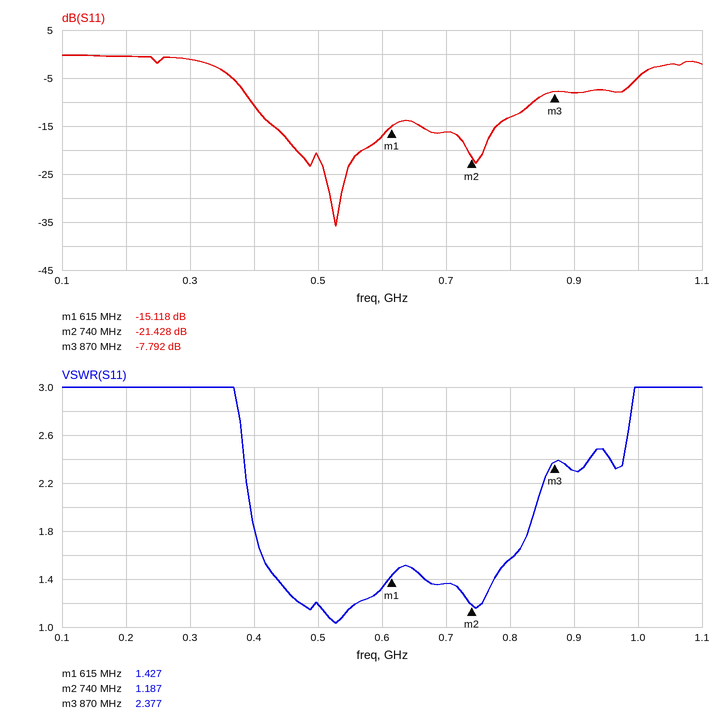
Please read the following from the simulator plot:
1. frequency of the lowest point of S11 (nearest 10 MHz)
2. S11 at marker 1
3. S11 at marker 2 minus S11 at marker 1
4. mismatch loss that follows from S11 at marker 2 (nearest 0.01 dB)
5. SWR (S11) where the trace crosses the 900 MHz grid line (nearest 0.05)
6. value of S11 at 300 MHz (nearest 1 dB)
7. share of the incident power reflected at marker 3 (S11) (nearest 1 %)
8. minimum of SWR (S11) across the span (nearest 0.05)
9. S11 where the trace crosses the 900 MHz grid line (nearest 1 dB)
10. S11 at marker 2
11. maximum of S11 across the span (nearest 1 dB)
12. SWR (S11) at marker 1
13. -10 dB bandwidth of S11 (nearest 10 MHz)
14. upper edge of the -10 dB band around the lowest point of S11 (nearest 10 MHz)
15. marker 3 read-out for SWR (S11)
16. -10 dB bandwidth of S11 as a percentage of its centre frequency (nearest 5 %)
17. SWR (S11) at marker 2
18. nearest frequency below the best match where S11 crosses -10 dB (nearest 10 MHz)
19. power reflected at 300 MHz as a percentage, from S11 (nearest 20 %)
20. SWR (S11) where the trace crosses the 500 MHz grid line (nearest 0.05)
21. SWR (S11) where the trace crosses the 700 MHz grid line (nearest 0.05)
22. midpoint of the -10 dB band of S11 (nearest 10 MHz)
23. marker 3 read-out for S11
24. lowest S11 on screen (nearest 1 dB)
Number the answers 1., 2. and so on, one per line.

1. 530 MHz
2. -15.118 dB
3. -6.310 dB
4. 0.03 dB
5. 2.30
6. -1 dB
7. 17 %
8. 1.05
9. -8 dB
10. -21.428 dB
11. 0 dB
12. 1.427
13. 440 MHz
14. 840 MHz
15. 2.377
16. 70 %
17. 1.187
18. 400 MHz
19. 80 %
20. 1.20
21. 1.35
22. 620 MHz
23. -7.792 dB
24. -36 dB
